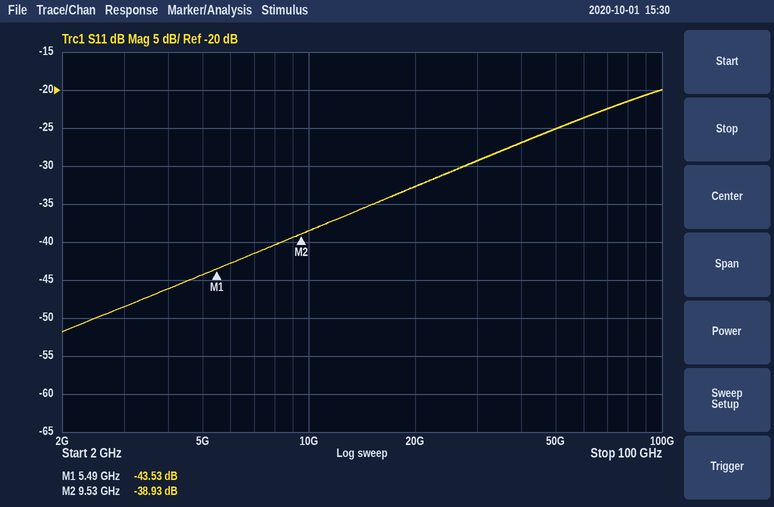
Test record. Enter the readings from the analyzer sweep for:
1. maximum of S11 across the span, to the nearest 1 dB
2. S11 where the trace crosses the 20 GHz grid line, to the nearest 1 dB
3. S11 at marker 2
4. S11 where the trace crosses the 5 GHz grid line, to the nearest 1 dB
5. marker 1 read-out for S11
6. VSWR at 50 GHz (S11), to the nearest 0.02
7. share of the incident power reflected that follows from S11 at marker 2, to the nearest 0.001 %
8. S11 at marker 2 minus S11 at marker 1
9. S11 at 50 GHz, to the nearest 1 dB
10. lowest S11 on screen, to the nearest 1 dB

-20 dB
-33 dB
-38.93 dB
-44 dB
-43.53 dB
1.12
0.013 %
4.60 dB
-25 dB
-52 dB
